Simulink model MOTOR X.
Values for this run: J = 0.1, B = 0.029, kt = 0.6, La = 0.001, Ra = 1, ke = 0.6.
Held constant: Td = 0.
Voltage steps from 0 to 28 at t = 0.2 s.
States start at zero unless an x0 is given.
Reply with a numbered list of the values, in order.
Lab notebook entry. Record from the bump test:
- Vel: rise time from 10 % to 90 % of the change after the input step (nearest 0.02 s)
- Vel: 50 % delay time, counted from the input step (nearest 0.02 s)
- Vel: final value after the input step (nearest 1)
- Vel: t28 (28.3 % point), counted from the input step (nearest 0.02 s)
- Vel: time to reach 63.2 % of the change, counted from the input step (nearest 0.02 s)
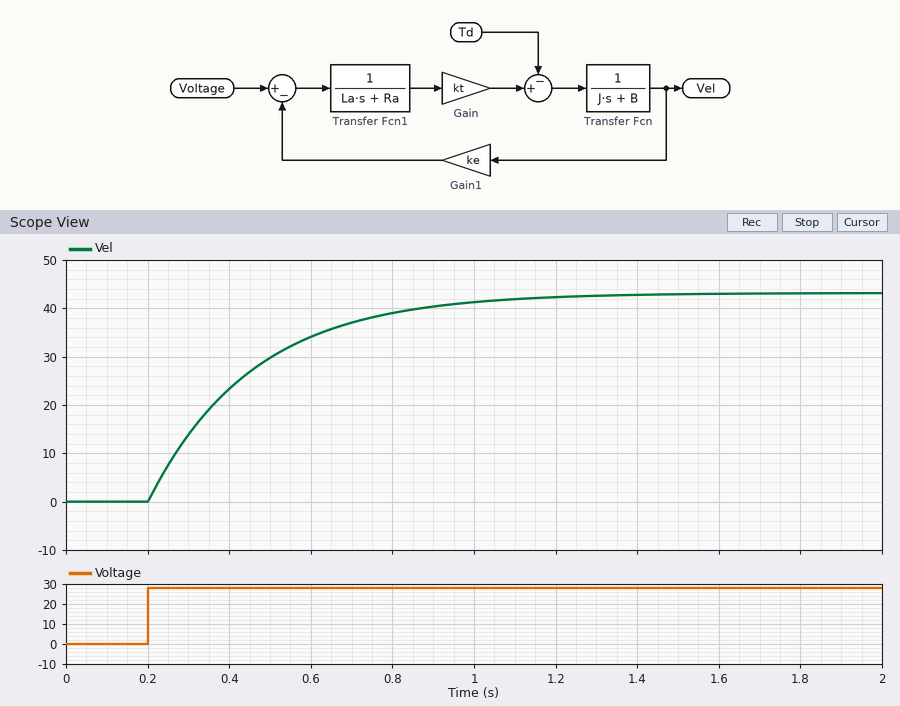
1. 0.56 s
2. 0.18 s
3. 43
4. 0.08 s
5. 0.26 s
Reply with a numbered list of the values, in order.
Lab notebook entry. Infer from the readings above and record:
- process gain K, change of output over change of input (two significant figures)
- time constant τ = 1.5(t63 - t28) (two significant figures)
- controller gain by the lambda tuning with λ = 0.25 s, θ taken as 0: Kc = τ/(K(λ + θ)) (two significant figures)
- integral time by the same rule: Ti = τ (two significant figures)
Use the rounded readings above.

1. 1.5
2. 0.27 s
3. 0.72
4. 0.27 s
